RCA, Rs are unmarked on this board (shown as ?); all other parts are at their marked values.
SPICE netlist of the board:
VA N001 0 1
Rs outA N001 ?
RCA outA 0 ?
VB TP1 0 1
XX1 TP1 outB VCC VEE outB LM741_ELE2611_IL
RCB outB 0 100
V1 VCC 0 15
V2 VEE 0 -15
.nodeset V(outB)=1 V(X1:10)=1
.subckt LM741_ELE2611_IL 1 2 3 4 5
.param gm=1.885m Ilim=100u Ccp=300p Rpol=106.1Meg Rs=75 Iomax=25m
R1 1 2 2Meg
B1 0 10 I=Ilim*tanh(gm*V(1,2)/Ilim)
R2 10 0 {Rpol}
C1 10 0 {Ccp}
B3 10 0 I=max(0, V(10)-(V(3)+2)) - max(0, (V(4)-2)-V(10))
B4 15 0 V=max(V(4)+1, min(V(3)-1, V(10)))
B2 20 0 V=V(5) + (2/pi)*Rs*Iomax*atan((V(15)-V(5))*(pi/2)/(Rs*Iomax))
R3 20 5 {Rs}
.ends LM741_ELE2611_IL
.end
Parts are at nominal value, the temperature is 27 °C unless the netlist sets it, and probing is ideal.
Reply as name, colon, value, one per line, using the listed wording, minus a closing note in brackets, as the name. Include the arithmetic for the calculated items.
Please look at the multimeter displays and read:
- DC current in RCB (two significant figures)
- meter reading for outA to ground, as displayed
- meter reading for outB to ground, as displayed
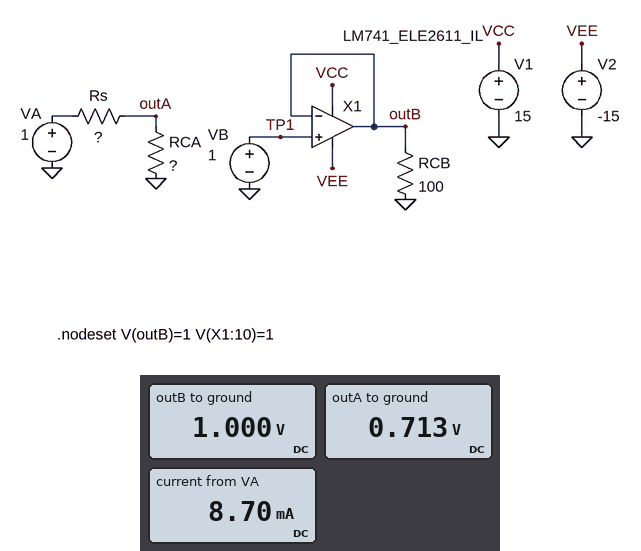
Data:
DC current in RCB: (1 V) / 100 Ω = 10 mA
meter reading for outA to ground, as displayed: 0.713 V
meter reading for outB to ground, as displayed: 1.000 V
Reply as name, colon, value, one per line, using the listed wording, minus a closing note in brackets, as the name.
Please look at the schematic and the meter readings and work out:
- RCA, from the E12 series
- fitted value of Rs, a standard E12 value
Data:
RCA, from the E12 series: 82 Ω
fitted value of Rs, a standard E12 value: 33 Ω
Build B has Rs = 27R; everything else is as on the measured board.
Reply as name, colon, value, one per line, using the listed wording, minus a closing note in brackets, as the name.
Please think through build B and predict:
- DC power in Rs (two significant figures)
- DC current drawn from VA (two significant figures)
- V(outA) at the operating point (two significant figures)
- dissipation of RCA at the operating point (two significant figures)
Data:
DC power in Rs: 2.3 mW
DC current drawn from VA: 9.2 mA
V(outA) at the operating point: 750 mV
dissipation of RCA at the operating point: 6.9 mW
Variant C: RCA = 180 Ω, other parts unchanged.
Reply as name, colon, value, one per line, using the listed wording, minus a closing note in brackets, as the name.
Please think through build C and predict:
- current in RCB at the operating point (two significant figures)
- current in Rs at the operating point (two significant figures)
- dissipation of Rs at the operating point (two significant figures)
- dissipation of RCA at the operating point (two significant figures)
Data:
current in RCB at the operating point: 10 mA
current in Rs at the operating point: 4.7 mA
dissipation of Rs at the operating point: 730 µW
dissipation of RCA at the operating point: 4.0 mW
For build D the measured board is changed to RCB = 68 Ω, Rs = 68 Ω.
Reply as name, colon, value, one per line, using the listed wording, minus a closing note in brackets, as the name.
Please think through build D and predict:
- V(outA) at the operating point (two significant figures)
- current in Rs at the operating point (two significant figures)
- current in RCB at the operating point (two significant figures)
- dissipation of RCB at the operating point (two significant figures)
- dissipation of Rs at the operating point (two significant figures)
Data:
V(outA) at the operating point: 550 mV
current in Rs at the operating point: 6.7 mA
current in RCB at the operating point: 15 mA
dissipation of RCB at the operating point: 15 mW
dissipation of Rs at the operating point: 3.0 mW
